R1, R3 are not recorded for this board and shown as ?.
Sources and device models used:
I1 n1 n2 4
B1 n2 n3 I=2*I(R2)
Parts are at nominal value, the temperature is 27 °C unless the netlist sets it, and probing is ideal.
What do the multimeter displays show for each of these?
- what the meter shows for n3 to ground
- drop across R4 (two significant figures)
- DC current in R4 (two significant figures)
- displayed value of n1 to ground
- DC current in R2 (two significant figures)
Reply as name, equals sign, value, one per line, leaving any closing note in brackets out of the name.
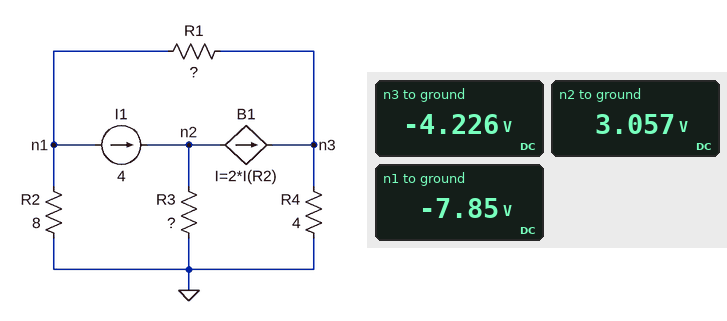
what the meter shows for n3 to ground = -4.226 V
drop across R4 = 4.2 V
DC current in R4 = 1.1 A
displayed value of n1 to ground = -7.85 V
DC current in R2 = 980 mA
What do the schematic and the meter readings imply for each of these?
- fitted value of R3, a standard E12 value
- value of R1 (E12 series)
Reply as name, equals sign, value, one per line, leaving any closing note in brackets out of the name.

fitted value of R3, a standard E12 value = 1.5 Ω
value of R1 = 1.2 Ω
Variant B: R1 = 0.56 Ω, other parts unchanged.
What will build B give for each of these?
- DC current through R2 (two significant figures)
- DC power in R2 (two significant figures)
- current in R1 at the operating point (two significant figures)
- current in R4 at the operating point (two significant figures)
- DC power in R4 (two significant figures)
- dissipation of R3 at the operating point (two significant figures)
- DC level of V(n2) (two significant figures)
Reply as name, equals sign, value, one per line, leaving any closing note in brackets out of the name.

DC current through R2 = 890 mA
DC power in R2 = 6.3 W
current in R1 at the operating point = 3.1 A
current in R4 at the operating point = 1.3 A
DC power in R4 = 7.2 W
dissipation of R3 at the operating point = 7.4 W
DC level of V(n2) = 3.3 V
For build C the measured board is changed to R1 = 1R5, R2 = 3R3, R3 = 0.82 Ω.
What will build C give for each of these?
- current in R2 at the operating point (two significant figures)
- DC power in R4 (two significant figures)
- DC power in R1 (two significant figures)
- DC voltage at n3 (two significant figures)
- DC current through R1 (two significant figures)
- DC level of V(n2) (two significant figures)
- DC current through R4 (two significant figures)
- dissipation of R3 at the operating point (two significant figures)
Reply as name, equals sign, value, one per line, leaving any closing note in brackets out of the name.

current in R2 at the operating point = 1.3 A
DC power in R4 = 20 mW
DC power in R1 = 11 W
DC voltage at n3 = -290 mV
DC current through R1 = 2.7 A
DC level of V(n2) = 1.1 V
DC current through R4 = 71 mA
dissipation of R3 at the operating point = 1.6 W
